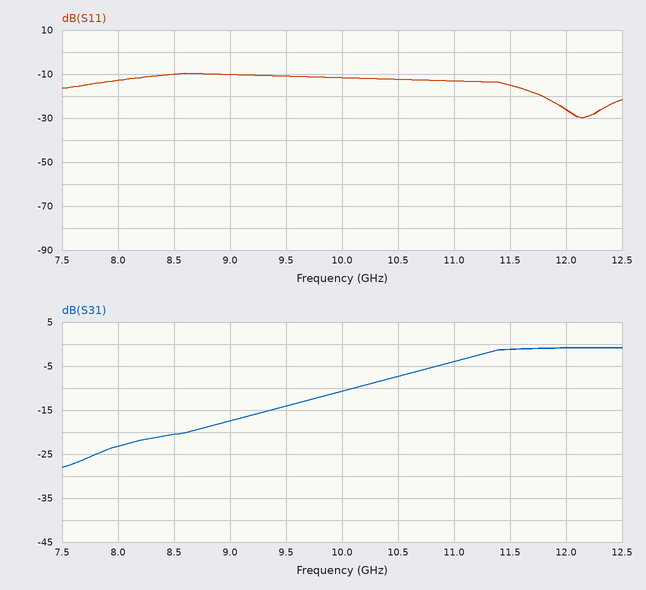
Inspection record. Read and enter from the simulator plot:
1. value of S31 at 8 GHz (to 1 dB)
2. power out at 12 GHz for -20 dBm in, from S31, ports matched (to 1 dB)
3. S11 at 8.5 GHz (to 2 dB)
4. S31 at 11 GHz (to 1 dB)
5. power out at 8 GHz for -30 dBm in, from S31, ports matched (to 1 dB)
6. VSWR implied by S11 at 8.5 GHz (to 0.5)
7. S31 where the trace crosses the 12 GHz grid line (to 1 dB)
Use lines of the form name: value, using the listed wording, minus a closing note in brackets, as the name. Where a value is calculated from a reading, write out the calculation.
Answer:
value of S31 at 8 GHz: -23 dB
power out at 12 GHz for -20 dBm in, from S31, ports matched: -20 dBm + (-1 dB) = -21 dBm
S11 at 8.5 GHz: -10 dB
S31 at 11 GHz: -4 dB
power out at 8 GHz for -30 dBm in, from S31, ports matched: -30 dBm + (-23 dB) = -53 dBm
VSWR implied by S11 at 8.5 GHz: |Γ| = 10^(-10/20) = 0.3162; VSWR = (1 + 0.3162)/(1 − 0.3162) ≈ 1.92, so 2.0 to the nearest 0.5
S31 where the trace crosses the 12 GHz grid line: -1 dB
